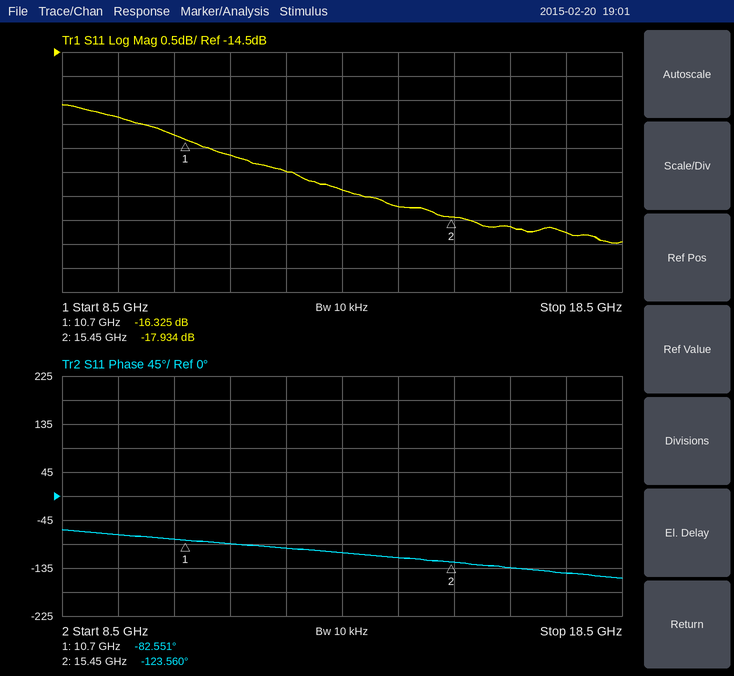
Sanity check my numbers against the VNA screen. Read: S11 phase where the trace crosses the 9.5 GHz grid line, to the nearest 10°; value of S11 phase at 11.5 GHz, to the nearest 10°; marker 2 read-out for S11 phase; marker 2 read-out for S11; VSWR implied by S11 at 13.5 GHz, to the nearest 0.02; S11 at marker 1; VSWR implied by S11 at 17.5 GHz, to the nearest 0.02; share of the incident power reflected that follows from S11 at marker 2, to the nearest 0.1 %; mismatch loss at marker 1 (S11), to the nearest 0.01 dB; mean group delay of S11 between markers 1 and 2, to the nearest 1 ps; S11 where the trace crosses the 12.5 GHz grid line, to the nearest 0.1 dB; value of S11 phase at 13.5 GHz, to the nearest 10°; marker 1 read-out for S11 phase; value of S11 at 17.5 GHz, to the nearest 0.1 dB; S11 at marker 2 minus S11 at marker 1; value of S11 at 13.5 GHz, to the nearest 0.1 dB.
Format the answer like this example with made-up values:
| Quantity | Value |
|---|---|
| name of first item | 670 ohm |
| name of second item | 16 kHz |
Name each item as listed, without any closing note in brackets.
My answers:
| Quantity | Value |
|---|---|
| S11 phase where the trace crosses the 9.5 GHz grid line, to the nearest 10° | -70° |
| value of S11 phase at 11.5 GHz, to the nearest 10° | -90° |
| marker 2 read-out for S11 phase | -123.560° |
| marker 2 read-out for S11 | -17.934 dB |
| VSWR implied by S11 at 13.5 GHz, to the nearest 0.02 | 1.32 |
| S11 at marker 1 | -16.325 dB |
| VSWR implied by S11 at 17.5 GHz, to the nearest 0.02 | 1.28 |
| share of the incident power reflected that follows from S11 at marker 2, to the nearest 0.1 % | 1.6 % |
| mismatch loss at marker 1 (S11), to the nearest 0.01 dB | 0.10 dB |
| mean group delay of S11 between markers 1 and 2, to the nearest 1 ps | 24 ps |
| S11 where the trace crosses the 12.5 GHz grid line, to the nearest 0.1 dB | -17.0 dB |
| value of S11 phase at 13.5 GHz, to the nearest 10° | -110° |
| marker 1 read-out for S11 phase | -82.551° |
| value of S11 at 17.5 GHz, to the nearest 0.1 dB | -18.3 dB |
| S11 at marker 2 minus S11 at marker 1 | -1.609 dB |
| value of S11 at 13.5 GHz, to the nearest 0.1 dB | -17.4 dB |
